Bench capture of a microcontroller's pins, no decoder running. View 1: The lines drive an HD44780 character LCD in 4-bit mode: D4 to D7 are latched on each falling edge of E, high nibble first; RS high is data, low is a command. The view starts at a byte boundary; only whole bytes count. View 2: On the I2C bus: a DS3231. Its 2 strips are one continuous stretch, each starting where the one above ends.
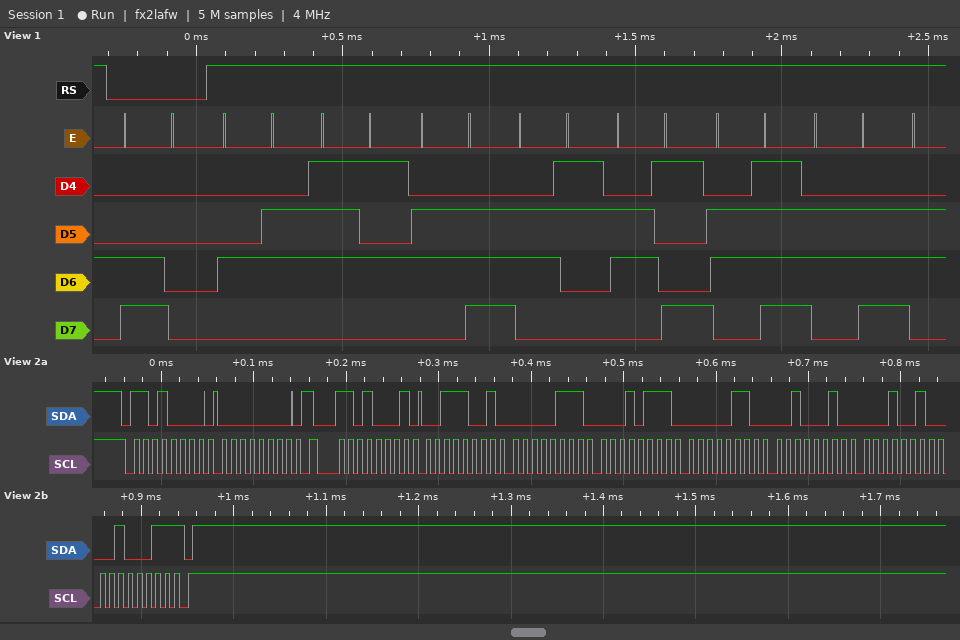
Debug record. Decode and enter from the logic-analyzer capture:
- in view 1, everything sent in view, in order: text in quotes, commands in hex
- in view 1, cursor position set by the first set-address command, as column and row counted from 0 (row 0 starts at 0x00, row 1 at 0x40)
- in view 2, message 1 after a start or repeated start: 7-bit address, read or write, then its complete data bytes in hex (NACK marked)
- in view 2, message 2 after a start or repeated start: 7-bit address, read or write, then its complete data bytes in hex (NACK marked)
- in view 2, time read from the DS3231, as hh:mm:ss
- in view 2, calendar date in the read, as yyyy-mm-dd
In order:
0xC0 "Funcion"
column 0, row 1
0x68 write: 00
0x68 read: 39 07 17 06 22 12 23 NACK
17:07:39
2023-12-22
